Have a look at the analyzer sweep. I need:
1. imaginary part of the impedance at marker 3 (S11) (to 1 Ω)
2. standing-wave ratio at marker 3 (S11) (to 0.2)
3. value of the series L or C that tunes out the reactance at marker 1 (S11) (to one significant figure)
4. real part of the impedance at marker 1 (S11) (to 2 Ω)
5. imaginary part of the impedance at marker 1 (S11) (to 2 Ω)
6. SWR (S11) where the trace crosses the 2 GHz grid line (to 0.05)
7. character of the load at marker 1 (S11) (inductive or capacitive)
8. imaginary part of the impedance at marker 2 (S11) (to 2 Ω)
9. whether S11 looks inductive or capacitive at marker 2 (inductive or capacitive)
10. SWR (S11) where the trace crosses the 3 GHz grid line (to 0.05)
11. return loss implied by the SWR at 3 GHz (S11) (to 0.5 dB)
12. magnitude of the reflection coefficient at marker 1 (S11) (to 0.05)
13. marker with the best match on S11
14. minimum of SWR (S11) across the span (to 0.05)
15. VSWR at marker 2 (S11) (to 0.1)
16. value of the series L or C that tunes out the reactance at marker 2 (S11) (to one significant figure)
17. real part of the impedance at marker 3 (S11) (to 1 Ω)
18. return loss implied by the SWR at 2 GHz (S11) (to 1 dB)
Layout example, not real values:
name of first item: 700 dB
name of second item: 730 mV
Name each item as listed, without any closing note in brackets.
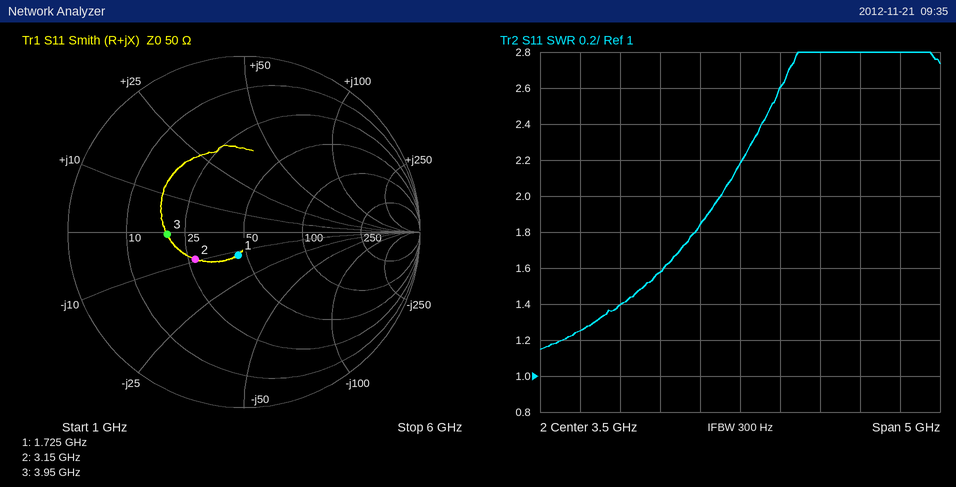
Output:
imaginary part of the impedance at marker 3 (S11): -1 Ω
standing-wave ratio at marker 3 (S11): 2.6
value of the series L or C that tunes out the reactance at marker 1 (S11): 1 nH
real part of the impedance at marker 1 (S11): 46 Ω
imaginary part of the impedance at marker 1 (S11): -12 Ω
SWR (S11) where the trace crosses the 2 GHz grid line: 1.40
character of the load at marker 1 (S11): capacitive
imaginary part of the impedance at marker 2 (S11): -10 Ω
whether S11 looks inductive or capacitive at marker 2: capacitive
SWR (S11) where the trace crosses the 3 GHz grid line: 1.85
return loss implied by the SWR at 3 GHz (S11): 10.5 dB
magnitude of the reflection coefficient at marker 1 (S11): 0.15
marker with the best match on S11: marker 1
minimum of SWR (S11) across the span: 1.15
VSWR at marker 2 (S11): 1.9
value of the series L or C that tunes out the reactance at marker 2 (S11): 500 pH
real part of the impedance at marker 3 (S11): 20 Ω
return loss implied by the SWR at 2 GHz (S11): 16 dB
